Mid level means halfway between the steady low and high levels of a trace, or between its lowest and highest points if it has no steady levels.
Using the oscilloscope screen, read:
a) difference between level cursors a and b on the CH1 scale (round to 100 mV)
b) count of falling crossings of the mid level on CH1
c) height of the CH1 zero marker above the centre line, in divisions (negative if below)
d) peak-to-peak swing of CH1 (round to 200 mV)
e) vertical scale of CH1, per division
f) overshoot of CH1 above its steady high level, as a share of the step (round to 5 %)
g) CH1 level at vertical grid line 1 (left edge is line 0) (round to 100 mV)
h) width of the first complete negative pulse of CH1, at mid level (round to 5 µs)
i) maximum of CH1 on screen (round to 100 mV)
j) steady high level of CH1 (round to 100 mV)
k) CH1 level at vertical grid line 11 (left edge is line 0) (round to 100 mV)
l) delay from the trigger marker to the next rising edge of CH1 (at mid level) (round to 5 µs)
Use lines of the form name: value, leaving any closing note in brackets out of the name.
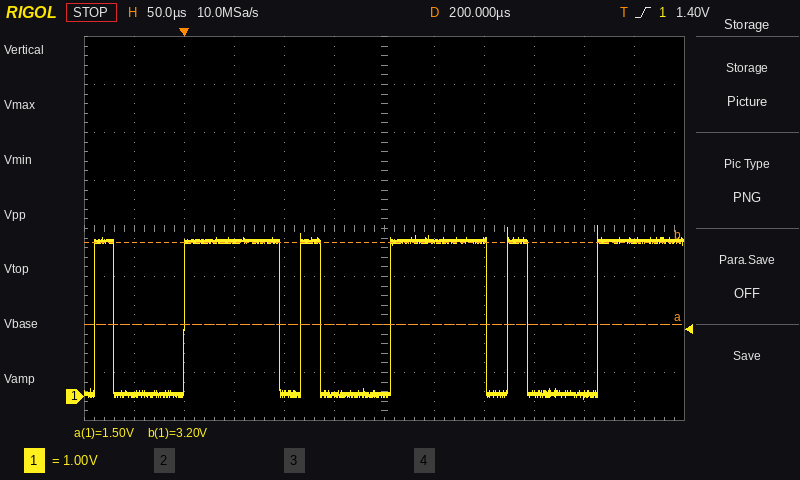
difference between level cursors a and b on the CH1 scale: 1.7 V
count of falling crossings of the mid level on CH1: 5
height of the CH1 zero marker above the centre line, in divisions: -3.5 div
peak-to-peak swing of CH1: 3.6 V
vertical scale of CH1, per division: 1 V
overshoot of CH1 above its steady high level, as a share of the step: 10 %
CH1 level at vertical grid line 1 (left edge is line 0): 100 mV
width of the first complete negative pulse of CH1, at mid level: 70 µs
maximum of CH1 on screen: 3.6 V
steady high level of CH1: 3.2 V
CH1 level at vertical grid line 11 (left edge is line 0): 3.2 V
delay from the trigger marker to the next rising edge of CH1 (at mid level): 115 µs
